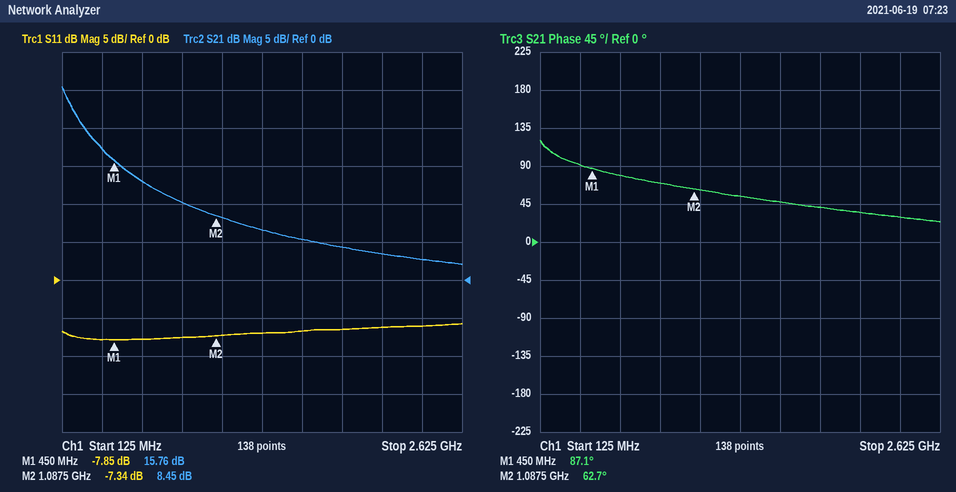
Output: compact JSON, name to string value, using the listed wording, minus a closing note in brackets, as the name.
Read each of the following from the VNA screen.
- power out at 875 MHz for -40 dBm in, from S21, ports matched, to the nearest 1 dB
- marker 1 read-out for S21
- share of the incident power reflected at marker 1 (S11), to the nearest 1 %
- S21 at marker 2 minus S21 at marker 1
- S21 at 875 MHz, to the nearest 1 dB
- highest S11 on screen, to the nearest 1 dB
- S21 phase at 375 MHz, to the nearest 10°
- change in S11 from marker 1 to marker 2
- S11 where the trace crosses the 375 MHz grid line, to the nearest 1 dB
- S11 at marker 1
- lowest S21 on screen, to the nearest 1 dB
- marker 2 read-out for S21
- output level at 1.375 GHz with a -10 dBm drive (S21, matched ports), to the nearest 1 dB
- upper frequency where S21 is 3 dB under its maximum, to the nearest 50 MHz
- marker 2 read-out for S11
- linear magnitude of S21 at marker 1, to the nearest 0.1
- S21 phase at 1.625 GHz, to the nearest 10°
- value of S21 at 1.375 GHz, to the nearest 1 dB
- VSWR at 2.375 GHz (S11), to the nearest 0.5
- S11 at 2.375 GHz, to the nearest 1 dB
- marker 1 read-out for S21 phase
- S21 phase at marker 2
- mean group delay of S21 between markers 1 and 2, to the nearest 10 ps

{"power out at 875 MHz for -40 dBm in, from S21, ports matched, to the nearest 1 dB": "-30 dBm", "marker 1 read-out for S21": "15.76 dB", "share of the incident power reflected at marker 1 (S11), to the nearest 1 %": "16 %", "S21 at marker 2 minus S21 at marker 1": "-7.31 dB", "S21 at 875 MHz, to the nearest 1 dB": "10 dB", "highest S11 on screen, to the nearest 1 dB": "-6 dB", "S21 phase at 375 MHz, to the nearest 10°": "90°", "change in S11 from marker 1 to marker 2": "0.51 dB", "S11 where the trace crosses the 375 MHz grid line, to the nearest 1 dB": "-8 dB", "S11 at marker 1": "-7.85 dB", "lowest S21 on screen, to the nearest 1 dB": "2 dB", "marker 2 read-out for S21": "8.45 dB", "output level at 1.375 GHz with a -10 dBm drive (S21, matched ports), to the nearest 1 dB": "-3 dBm", "upper frequency where S21 is 3 dB under its maximum, to the nearest 50 MHz": "200 MHz", "marker 2 read-out for S11": "-7.34 dB", "linear magnitude of S21 at marker 1, to the nearest 0.1": "6.1", "S21 phase at 1.625 GHz, to the nearest 10°": "50°", "value of S21 at 1.375 GHz, to the nearest 1 dB": "7 dB", "VSWR at 2.375 GHz (S11), to the nearest 0.5": "3.0", "S11 at 2.375 GHz, to the nearest 1 dB": "-6 dB", "marker 1 read-out for S21 phase": "87.1°", "S21 phase at marker 2": "62.7°", "mean group delay of S21 between markers 1 and 2, to the nearest 10 ps": "110 ps"}
